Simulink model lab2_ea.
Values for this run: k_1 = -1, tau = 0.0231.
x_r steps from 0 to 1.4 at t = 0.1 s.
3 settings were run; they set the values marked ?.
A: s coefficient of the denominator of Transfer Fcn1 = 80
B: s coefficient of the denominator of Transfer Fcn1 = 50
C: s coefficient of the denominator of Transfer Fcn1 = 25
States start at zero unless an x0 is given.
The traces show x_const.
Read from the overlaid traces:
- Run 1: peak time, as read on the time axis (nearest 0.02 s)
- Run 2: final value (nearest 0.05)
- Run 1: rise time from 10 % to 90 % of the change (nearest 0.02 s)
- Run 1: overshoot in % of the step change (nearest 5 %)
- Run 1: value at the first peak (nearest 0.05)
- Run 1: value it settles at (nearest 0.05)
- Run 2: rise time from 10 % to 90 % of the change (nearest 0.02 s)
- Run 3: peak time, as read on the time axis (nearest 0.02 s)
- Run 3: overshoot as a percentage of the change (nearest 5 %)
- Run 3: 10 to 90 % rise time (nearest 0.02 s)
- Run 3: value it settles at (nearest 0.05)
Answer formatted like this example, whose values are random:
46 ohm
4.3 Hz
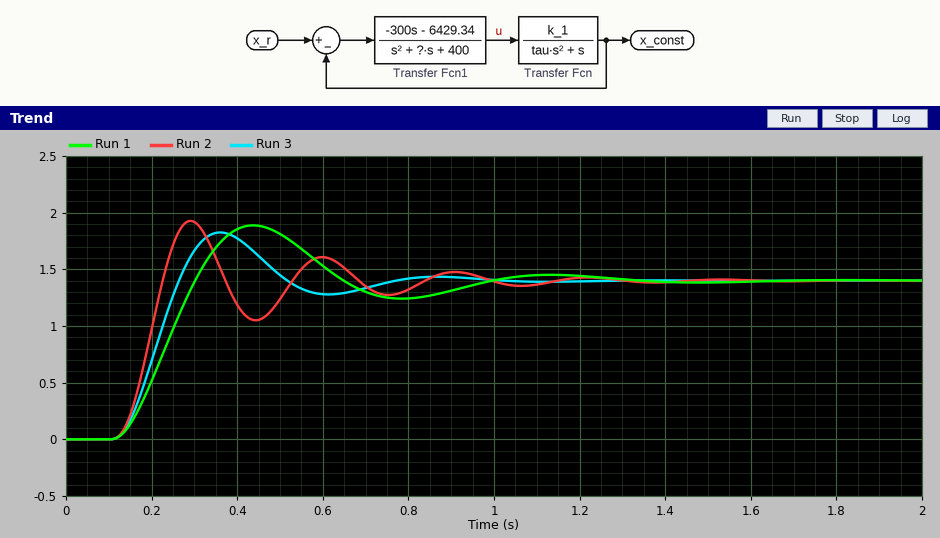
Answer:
0.44 s
1.40
0.14 s
35 %
1.90
1.40
0.08 s
0.36 s
30 %
0.10 s
1.40
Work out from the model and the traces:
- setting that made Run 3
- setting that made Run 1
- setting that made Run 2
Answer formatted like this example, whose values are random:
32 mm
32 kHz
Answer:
B
A
C
